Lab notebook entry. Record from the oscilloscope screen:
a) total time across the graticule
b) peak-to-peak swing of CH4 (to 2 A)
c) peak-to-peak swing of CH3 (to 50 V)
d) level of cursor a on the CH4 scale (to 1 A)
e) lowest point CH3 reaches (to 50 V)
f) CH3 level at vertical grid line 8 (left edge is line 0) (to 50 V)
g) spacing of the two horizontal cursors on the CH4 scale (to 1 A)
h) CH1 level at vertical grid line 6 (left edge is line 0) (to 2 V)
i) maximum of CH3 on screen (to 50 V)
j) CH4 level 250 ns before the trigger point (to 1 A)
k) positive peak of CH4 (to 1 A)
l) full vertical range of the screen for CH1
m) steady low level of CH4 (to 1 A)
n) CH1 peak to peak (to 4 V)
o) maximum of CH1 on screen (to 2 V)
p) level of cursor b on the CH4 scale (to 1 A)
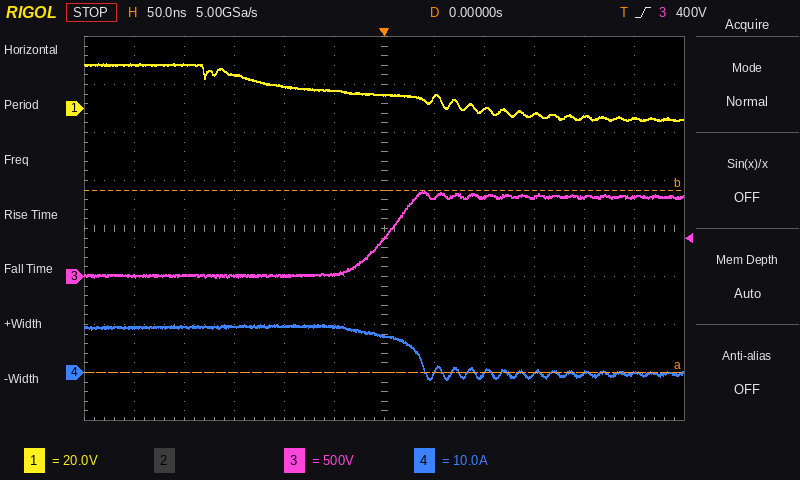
600 ns
12 A
900 V
0 A
0 V
850 V
38 A
6 V
900 V
9 A
10 A
160 V
0 A
24 V
18 V
38 A
